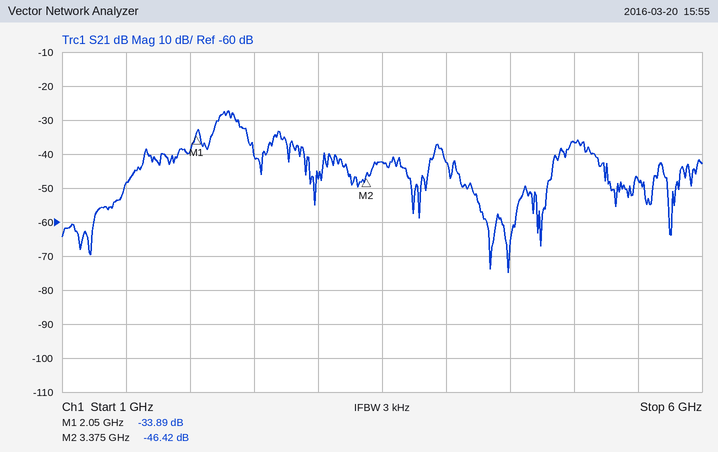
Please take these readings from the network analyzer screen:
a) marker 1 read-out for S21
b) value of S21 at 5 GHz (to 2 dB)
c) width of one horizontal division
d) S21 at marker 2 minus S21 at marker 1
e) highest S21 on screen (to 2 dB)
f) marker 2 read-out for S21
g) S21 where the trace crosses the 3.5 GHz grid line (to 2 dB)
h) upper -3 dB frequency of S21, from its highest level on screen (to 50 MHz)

-33.89 dB
-36 dB
500 MHz
-12.53 dB
-28 dB
-46.42 dB
-42 dB
2.35 GHz
